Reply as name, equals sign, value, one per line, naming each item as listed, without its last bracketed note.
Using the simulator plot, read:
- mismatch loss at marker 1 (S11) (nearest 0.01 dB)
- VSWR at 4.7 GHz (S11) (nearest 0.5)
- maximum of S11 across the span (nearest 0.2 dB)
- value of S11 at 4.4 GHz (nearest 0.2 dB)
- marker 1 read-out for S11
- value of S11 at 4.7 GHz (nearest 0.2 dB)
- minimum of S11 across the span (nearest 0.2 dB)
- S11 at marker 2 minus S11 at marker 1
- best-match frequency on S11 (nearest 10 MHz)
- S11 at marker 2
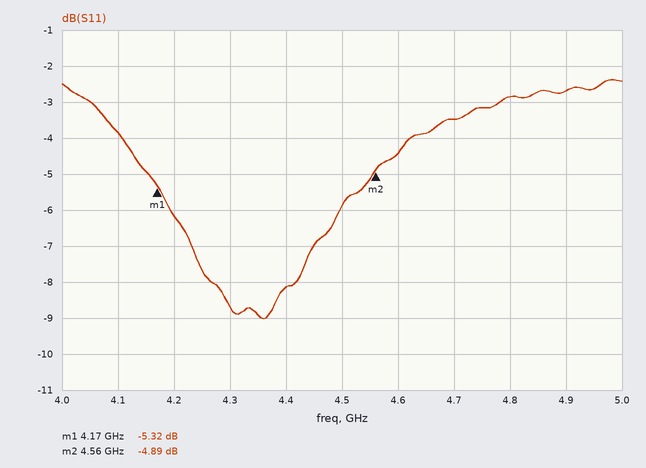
mismatch loss at marker 1 (S11) = 1.51 dB
VSWR at 4.7 GHz (S11) = 5.0
maximum of S11 across the span = -2.4 dB
value of S11 at 4.4 GHz = -8.2 dB
marker 1 read-out for S11 = -5.32 dB
value of S11 at 4.7 GHz = -3.4 dB
minimum of S11 across the span = -9.0 dB
S11 at marker 2 minus S11 at marker 1 = 0.43 dB
best-match frequency on S11 = 4.36 GHz
S11 at marker 2 = -4.89 dB
